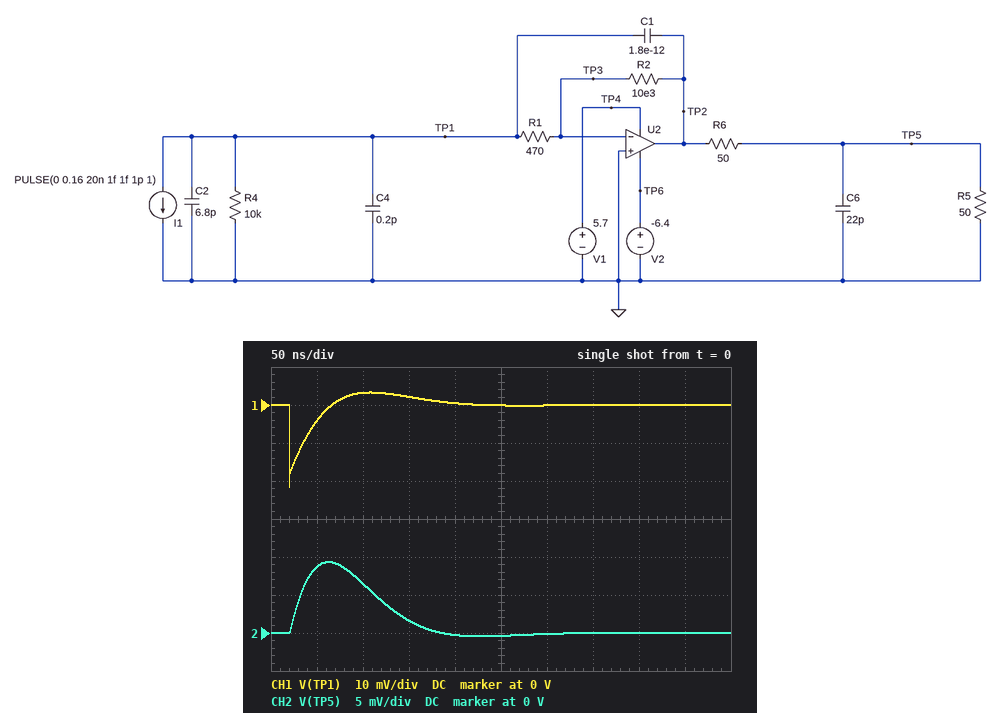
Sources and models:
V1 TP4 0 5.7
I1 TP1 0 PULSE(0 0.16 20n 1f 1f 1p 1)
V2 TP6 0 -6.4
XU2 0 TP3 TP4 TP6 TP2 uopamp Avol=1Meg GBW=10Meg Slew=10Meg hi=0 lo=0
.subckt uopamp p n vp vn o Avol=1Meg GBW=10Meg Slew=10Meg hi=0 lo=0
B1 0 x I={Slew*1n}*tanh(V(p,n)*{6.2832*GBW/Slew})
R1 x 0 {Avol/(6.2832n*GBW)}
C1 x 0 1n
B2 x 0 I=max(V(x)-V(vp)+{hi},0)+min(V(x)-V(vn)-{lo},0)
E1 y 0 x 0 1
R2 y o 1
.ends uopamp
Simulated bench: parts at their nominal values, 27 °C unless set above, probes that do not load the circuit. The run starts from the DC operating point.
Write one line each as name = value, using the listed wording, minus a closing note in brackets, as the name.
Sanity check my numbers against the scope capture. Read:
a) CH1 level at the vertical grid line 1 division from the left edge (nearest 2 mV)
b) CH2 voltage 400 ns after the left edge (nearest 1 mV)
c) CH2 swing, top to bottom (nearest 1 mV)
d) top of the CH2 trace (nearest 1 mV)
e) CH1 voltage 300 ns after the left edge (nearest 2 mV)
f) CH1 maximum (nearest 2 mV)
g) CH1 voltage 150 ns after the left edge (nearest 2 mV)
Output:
CH1 level at the vertical grid line 1 division from the left edge = -4 mV
CH2 voltage 400 ns after the left edge = 0 V
CH2 swing, top to bottom = 10 mV
top of the CH2 trace = 9 mV
CH1 voltage 300 ns after the left edge = 0 V
CH1 maximum = 4 mV
CH1 voltage 150 ns after the left edge = 2 mV
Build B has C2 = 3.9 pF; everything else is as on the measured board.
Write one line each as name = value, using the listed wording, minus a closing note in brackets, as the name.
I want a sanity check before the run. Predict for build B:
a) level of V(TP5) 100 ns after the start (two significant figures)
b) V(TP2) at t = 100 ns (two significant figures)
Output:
level of V(TP5) 100 ns after the start = 5.2 mV
V(TP2) at t = 100 ns = 10 mV
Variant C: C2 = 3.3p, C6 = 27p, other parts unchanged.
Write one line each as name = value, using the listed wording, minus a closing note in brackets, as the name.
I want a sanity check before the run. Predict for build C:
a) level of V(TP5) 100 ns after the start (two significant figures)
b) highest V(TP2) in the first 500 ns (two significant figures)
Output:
level of V(TP5) 100 ns after the start = 4.9 mV
highest V(TP2) in the first 500 ns = 21 mV
